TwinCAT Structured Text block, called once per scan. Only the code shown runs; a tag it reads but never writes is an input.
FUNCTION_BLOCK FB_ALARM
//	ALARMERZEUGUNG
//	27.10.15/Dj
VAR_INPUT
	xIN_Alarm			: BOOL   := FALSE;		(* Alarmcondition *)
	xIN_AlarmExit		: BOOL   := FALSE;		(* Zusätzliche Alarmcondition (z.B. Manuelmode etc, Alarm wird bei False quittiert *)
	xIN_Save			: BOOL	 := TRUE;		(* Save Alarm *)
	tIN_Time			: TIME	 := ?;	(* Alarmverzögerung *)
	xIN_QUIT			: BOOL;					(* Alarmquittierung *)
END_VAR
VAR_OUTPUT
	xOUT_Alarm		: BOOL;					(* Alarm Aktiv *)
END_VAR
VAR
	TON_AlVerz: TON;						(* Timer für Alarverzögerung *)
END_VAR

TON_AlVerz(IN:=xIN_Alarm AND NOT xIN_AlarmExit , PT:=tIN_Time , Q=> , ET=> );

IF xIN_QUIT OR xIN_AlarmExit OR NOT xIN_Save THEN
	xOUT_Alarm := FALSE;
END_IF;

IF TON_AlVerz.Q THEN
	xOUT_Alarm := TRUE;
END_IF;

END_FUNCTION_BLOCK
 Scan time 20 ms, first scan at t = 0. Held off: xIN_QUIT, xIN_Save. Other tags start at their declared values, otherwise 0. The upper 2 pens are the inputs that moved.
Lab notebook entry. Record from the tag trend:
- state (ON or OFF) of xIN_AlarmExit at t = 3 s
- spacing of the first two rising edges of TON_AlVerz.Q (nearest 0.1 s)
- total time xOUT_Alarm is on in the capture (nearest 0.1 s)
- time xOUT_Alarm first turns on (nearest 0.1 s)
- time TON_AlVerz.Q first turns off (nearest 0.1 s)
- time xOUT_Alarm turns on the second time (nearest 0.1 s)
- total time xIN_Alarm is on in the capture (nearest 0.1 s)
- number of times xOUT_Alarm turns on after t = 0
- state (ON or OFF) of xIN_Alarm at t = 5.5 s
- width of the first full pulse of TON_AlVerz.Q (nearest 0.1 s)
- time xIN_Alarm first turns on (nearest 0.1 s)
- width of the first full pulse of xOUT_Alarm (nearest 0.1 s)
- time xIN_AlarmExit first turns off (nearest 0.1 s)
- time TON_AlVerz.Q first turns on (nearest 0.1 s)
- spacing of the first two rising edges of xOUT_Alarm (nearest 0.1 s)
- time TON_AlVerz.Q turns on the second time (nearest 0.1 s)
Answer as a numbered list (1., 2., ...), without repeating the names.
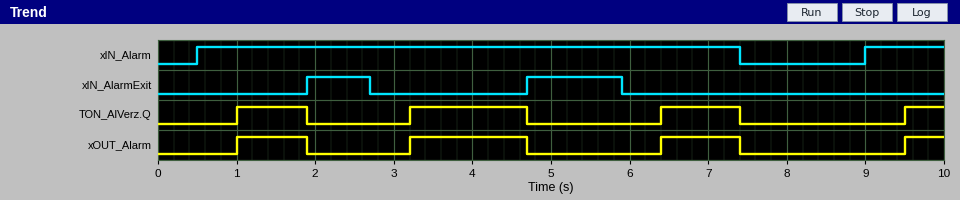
1. OFF
2. 2.2 s
3. 3.9 s
4. 1.0 s
5. 1.9 s
6. 3.2 s
7. 7.9 s
8. 4
9. ON
10. 0.9 s
11. 0.5 s
12. 0.9 s
13. 2.7 s
14. 1.0 s
15. 2.2 s
16. 3.2 s
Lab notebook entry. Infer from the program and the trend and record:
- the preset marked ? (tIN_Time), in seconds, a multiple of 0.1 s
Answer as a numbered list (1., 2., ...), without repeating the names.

1. 0.5 s
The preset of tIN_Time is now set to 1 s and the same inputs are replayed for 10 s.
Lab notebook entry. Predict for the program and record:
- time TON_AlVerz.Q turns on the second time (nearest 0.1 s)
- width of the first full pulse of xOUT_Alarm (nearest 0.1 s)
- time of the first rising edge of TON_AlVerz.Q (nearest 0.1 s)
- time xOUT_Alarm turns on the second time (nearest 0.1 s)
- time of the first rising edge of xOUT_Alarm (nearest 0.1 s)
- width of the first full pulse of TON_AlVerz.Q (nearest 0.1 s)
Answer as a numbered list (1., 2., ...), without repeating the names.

1. 3.7 s
2. 0.4 s
3. 1.5 s
4. 3.7 s
5. 1.5 s
6. 0.4 s
